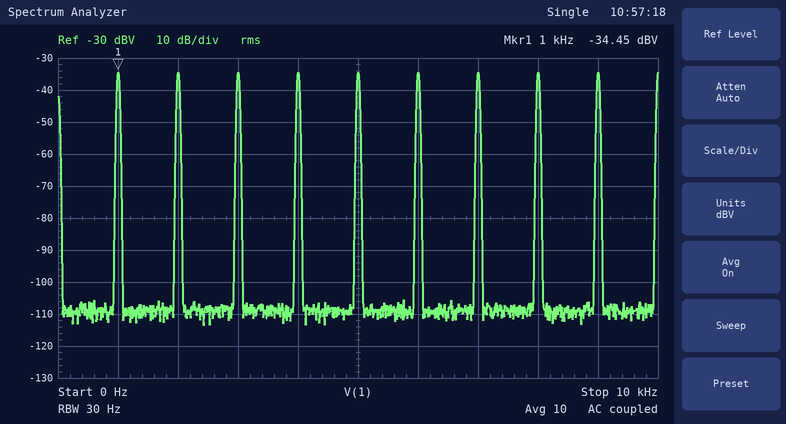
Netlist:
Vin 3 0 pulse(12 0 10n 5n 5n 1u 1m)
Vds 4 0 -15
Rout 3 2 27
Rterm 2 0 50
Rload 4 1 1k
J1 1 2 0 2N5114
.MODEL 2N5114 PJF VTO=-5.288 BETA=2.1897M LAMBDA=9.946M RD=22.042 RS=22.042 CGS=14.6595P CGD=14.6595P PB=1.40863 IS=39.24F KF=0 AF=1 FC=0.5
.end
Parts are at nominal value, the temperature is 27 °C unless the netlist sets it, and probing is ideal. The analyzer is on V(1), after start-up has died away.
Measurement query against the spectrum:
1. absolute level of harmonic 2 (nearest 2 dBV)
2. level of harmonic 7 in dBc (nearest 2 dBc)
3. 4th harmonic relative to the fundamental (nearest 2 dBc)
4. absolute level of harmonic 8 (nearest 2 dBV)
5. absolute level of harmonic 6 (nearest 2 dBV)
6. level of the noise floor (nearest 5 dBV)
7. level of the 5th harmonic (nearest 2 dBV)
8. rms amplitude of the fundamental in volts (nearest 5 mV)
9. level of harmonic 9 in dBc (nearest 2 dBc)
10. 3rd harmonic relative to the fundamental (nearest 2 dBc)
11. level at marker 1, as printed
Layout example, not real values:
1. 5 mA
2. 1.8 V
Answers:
1. -34 dBV
2. 0 dBc
3. 0 dBc
4. -34 dBV
5. -34 dBV
6. -110 dBV
7. -34 dBV
8. 20 mV
9. 0 dBc
10. 0 dBc
11. -34.45 dBV
